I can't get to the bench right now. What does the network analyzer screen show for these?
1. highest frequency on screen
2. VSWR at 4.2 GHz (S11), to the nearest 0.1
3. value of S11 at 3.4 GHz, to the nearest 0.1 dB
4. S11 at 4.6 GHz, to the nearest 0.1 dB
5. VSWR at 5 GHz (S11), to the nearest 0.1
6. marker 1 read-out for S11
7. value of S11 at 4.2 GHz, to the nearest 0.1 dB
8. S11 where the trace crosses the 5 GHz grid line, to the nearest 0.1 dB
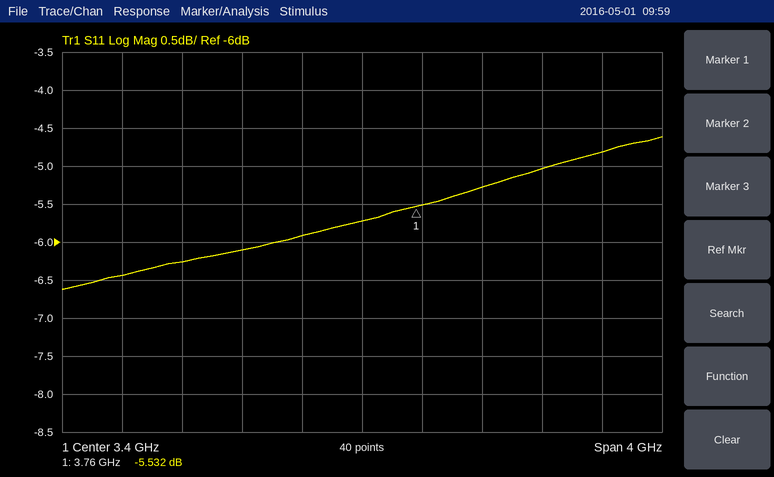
5.4 GHz
3.4
-5.7 dB
-5.0 dB
3.7
-5.532 dB
-5.3 dB
-4.8 dB
